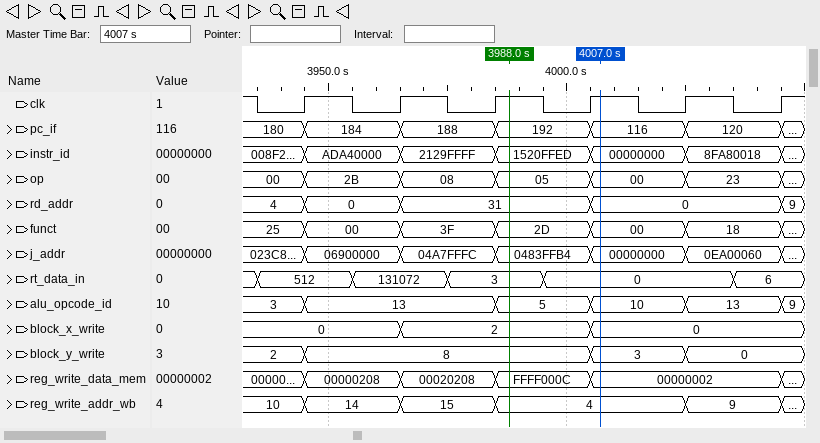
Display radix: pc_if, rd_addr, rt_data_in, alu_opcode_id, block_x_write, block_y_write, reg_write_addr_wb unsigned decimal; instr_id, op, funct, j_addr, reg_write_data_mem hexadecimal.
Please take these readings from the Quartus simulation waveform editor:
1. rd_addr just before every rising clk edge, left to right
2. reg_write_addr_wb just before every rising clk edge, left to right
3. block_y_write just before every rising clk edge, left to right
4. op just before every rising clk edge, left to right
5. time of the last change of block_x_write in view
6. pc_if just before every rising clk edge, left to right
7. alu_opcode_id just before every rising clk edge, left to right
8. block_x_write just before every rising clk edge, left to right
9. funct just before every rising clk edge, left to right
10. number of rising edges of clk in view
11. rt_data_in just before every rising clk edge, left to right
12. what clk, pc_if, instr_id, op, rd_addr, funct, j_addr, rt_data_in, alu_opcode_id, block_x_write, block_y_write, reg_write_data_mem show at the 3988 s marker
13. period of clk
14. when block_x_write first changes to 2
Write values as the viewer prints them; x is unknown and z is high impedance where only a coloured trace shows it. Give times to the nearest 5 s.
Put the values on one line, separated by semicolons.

4, 0, 31, 31, 0, 0; 10, 14, 15, 4, 4, 9; 2, 8, 8, 8, 3, 0; 00, 2B, 08, 05, 00, 23; 4005 s; 180, 184, 188, 192, 116, 120; 3, 13, 13, 5, 10, 13; 0, 0, 2, 2, 0, 0; 25, 00, 3F, 2D, 00, 18; 6; 512, 131072, 3, 0, 0, 6; clk=1, pc_if=192, instr_id=1520FFED, op=05, rd_addr=31, funct=2D, j_addr=0483FFB4, rt_data_in=3, alu_opcode_id=5, block_x_write=2, block_y_write=8, reg_write_data_mem=FFFF000C; 20 s; 3965 s
